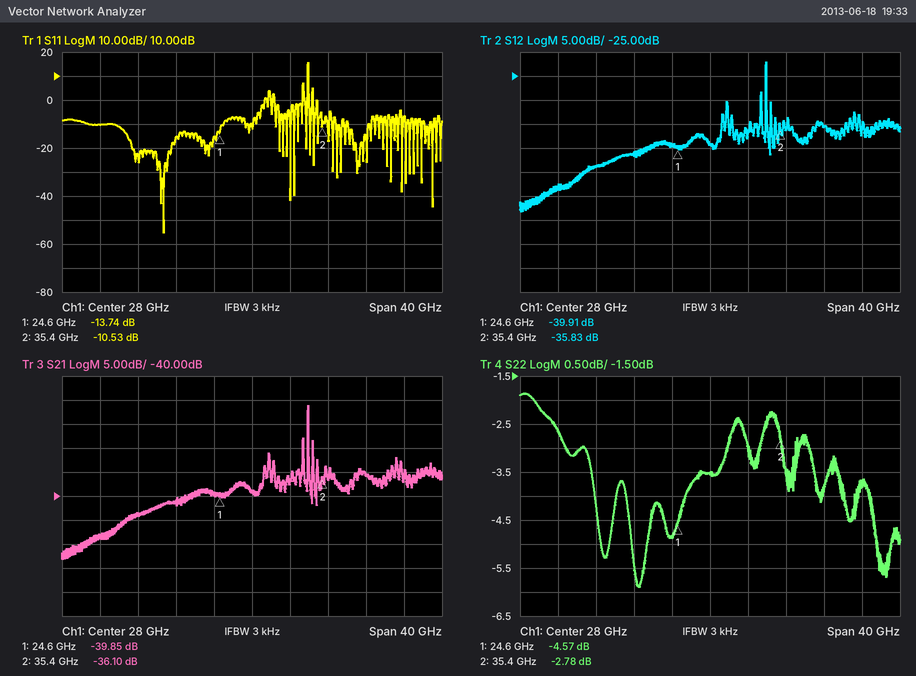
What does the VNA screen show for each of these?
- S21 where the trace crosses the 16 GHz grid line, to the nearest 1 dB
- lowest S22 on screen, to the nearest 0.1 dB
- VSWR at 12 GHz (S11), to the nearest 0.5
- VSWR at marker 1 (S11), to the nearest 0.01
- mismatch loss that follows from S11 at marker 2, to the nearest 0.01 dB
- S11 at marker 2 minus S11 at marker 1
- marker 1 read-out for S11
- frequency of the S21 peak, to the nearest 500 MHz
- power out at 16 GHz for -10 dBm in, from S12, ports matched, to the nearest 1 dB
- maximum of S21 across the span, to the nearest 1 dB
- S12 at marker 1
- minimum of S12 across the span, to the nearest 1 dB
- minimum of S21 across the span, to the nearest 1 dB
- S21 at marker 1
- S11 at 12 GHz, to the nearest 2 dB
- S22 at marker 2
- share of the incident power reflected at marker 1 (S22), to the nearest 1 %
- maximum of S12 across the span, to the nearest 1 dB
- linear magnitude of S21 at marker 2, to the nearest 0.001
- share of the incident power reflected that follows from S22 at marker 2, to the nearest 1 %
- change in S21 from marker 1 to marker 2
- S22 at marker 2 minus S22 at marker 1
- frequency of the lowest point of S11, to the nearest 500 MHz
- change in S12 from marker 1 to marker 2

-44 dB
-5.9 dB
2.0
1.52
0.40 dB
3.21 dB
-13.74 dB
34.0 GHz
-54 dBm
-21 dB
-39.91 dB
-53 dB
-53 dB
-39.85 dB
-10 dB
-2.78 dB
35 %
-22 dB
0.016
53 %
3.75 dB
1.79 dB
18.5 GHz
4.08 dB
